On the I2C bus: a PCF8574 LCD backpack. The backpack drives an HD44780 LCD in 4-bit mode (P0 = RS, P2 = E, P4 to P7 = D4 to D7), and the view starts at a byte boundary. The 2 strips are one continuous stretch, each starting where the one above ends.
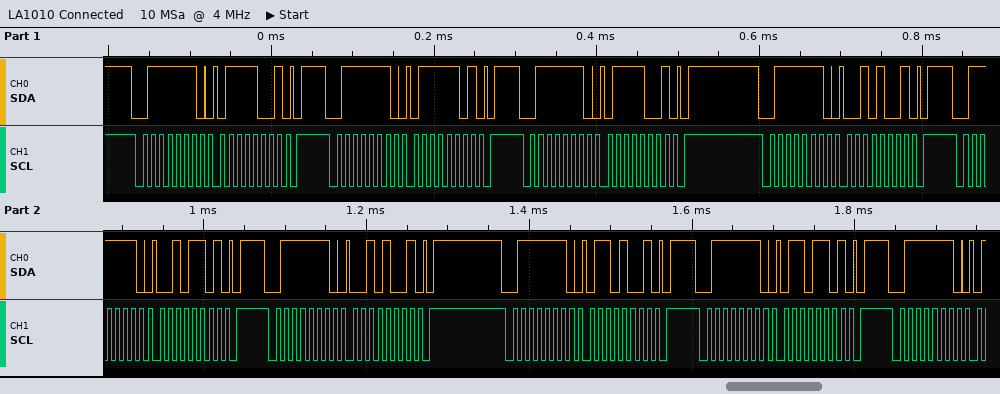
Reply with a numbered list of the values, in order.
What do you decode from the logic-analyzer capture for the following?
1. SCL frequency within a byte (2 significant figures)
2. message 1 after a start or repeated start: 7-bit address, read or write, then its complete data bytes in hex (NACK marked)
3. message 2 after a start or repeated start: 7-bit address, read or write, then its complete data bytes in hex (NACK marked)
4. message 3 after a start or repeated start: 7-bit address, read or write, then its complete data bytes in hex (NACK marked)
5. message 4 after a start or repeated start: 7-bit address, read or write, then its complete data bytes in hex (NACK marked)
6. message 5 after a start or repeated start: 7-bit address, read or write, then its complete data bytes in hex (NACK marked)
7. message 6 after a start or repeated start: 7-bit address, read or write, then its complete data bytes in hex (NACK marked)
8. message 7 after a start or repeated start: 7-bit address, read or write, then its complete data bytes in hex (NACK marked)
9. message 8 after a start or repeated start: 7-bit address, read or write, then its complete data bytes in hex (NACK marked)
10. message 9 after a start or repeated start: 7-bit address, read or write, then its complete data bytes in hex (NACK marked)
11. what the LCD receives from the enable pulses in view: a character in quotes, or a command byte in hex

1. 100 kHz
2. 0x3F write: 79
3. 0x3F write: 7D
4. 0x3F write: 79
5. 0x3F write: 29
6. 0x3F write: 2D
7. 0x3F write: 29
8. 0x3F write: 69
9. 0x3F write: 6D
10. 0x3F write
11. 'r'
